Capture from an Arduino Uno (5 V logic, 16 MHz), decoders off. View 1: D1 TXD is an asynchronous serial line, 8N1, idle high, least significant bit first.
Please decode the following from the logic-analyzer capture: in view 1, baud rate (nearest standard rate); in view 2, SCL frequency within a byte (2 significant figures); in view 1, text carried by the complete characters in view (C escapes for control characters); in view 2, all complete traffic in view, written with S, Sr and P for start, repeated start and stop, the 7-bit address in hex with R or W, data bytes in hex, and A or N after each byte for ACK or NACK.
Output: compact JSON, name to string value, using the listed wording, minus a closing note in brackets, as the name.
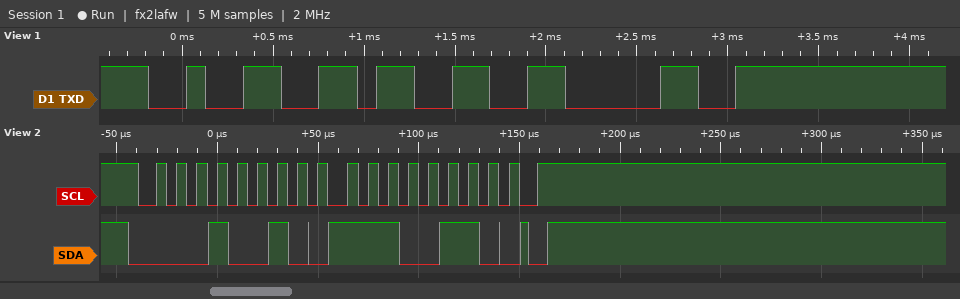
{"in view 1, baud rate": "9600 baud", "in view 2, SCL frequency within a byte": "100 kHz", "in view 1, text carried by the complete characters in view": "\"230\"", "in view 2, all complete traffic in view, written with S, Sr and P for start, repeated start and stop, the 7-bit address in hex with R or W, data bytes in hex, and A or N after each byte for ACK or NACK": "S 09W A E6 A P"}
